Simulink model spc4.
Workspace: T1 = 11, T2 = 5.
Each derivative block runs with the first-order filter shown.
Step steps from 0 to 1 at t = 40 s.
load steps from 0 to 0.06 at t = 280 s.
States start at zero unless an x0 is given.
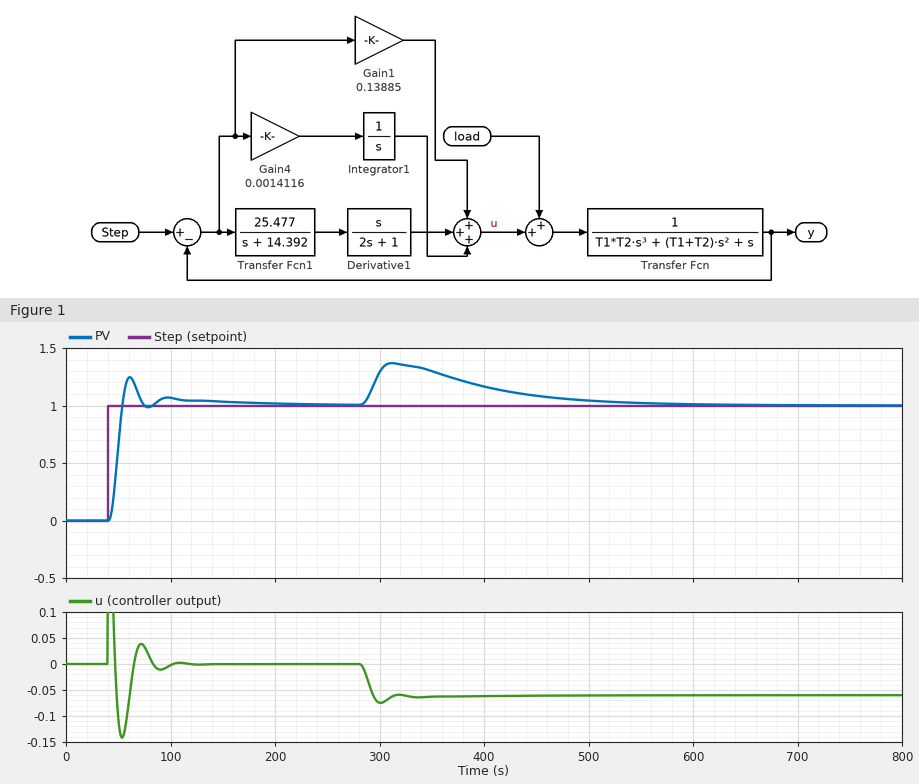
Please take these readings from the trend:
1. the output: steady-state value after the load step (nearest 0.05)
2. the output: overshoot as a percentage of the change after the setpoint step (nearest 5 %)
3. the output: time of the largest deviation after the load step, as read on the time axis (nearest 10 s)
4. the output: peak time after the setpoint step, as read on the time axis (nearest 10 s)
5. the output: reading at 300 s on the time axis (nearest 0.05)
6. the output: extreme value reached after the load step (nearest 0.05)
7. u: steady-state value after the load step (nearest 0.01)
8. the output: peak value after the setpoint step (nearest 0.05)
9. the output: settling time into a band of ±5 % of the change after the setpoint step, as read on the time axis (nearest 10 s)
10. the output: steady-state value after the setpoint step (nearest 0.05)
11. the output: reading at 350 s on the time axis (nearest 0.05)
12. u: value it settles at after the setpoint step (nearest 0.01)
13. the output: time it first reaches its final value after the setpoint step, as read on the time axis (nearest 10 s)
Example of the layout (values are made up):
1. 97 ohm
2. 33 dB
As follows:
1. 1.00
2. 25 %
3. 310 s
4. 60 s
5. 1.30
6. 1.35
7. -0.06
8. 1.25
9. 110 s
10. 1.00
11. 1.30
12. 0.00
13. 50 s
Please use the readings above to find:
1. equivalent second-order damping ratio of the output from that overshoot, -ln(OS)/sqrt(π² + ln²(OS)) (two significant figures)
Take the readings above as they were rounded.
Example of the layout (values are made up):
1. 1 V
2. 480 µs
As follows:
1. 0.40
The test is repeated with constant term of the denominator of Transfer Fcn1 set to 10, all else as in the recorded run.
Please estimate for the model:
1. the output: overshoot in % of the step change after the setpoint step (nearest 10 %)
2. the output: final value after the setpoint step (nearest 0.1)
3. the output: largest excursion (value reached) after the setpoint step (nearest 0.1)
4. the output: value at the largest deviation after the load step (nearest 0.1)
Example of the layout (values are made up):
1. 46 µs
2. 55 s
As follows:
1. 30 %
2. 1.0
3. 1.3
4. 1.3
